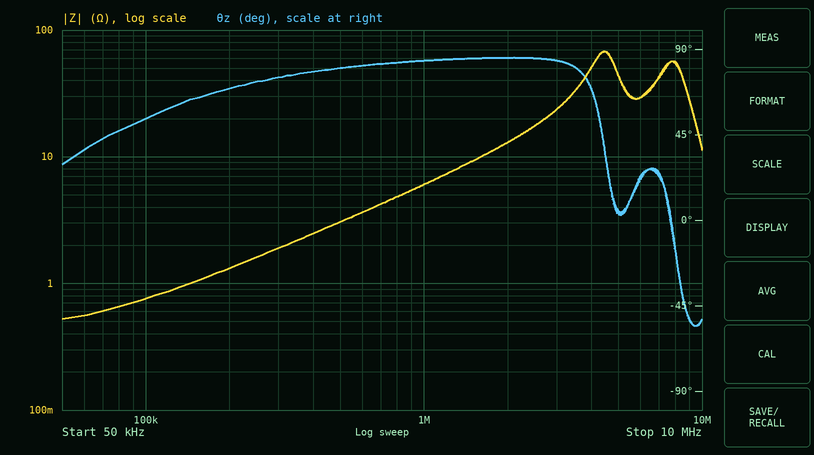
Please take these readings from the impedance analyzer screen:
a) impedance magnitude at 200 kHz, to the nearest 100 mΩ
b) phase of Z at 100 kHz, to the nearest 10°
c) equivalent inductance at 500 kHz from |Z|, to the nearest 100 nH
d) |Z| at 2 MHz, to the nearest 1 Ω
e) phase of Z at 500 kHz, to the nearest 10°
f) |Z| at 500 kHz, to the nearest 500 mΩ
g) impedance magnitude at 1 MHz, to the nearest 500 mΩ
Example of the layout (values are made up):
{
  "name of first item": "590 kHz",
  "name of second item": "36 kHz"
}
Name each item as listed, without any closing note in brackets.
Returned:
{
  "impedance magnitude at 200 kHz, to the nearest 100 mΩ": "1.3 Ω",
  "phase of Z at 100 kHz, to the nearest 10°": "50°",
  "equivalent inductance at 500 kHz from |Z|, to the nearest 100 nH": "1.0 µH",
  "|Z| at 2 MHz, to the nearest 1 Ω": "13 Ω",
  "phase of Z at 500 kHz, to the nearest 10°": "80°",
  "|Z| at 500 kHz, to the nearest 500 mΩ": "3.0 Ω",
  "impedance magnitude at 1 MHz, to the nearest 500 mΩ": "6.0 Ω"
}
